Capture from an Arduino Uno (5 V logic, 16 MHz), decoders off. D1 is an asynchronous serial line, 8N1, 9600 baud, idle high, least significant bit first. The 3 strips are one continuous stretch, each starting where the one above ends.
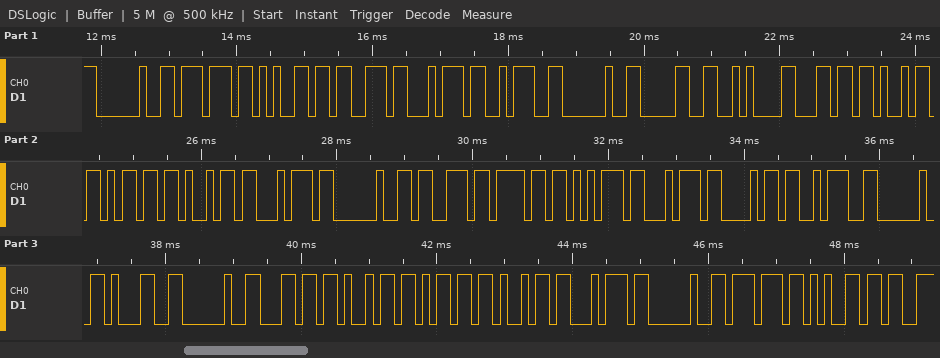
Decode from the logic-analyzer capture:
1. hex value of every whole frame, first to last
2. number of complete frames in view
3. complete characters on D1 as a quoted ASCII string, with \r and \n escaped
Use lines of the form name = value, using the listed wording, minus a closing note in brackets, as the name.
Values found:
hex value of every whole frame, first to last = 20 77 65 73 74 3A 20 30 0A 6C 69 6D 69 74 20 73 6F 75 74 68 3A 20 31 20 6C 69 6D 69 74 20 77 65
number of complete frames in view = 32
complete characters on D1 as a quoted ASCII string, with \r and \n escaped = " west: 0\nlimit south: 1 limit we"
